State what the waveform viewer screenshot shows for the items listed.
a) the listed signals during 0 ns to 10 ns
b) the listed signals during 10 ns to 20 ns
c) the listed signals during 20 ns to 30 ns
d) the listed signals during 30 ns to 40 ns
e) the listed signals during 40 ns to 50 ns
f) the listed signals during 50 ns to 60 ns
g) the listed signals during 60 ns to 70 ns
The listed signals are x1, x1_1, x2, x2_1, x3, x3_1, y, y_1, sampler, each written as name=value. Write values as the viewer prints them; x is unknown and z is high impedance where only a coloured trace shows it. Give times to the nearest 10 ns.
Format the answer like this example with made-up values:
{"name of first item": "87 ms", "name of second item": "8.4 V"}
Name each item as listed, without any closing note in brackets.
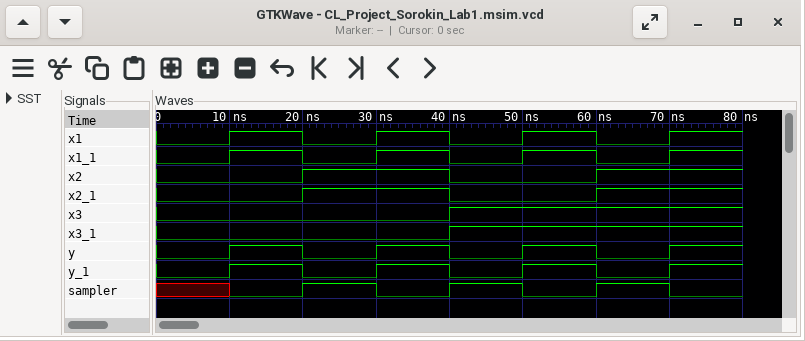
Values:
{"the listed signals during 0 ns to 10 ns": "x1=0, x1_1=0, x2=0, x2_1=0, x3=0, x3_1=0, y=0, y_1=0, sampler=x", "the listed signals during 10 ns to 20 ns": "x1=1, x1_1=1, x2=0, x2_1=0, x3=0, x3_1=0, y=1, y_1=1, sampler=0", "the listed signals during 20 ns to 30 ns": "x1=0, x1_1=0, x2=1, x2_1=1, x3=0, x3_1=0, y=0, y_1=0, sampler=1", "the listed signals during 30 ns to 40 ns": "x1=1, x1_1=1, x2=1, x2_1=1, x3=0, x3_1=0, y=1, y_1=1, sampler=0", "the listed signals during 40 ns to 50 ns": "x1=0, x1_1=0, x2=0, x2_1=0, x3=1, x3_1=1, y=0, y_1=0, sampler=1", "the listed signals during 50 ns to 60 ns": "x1=1, x1_1=1, x2=0, x2_1=0, x3=1, x3_1=1, y=1, y_1=1, sampler=0", "the listed signals during 60 ns to 70 ns": "x1=0, x1_1=0, x2=1, x2_1=1, x3=1, x3_1=1, y=0, y_1=0, sampler=1"}
